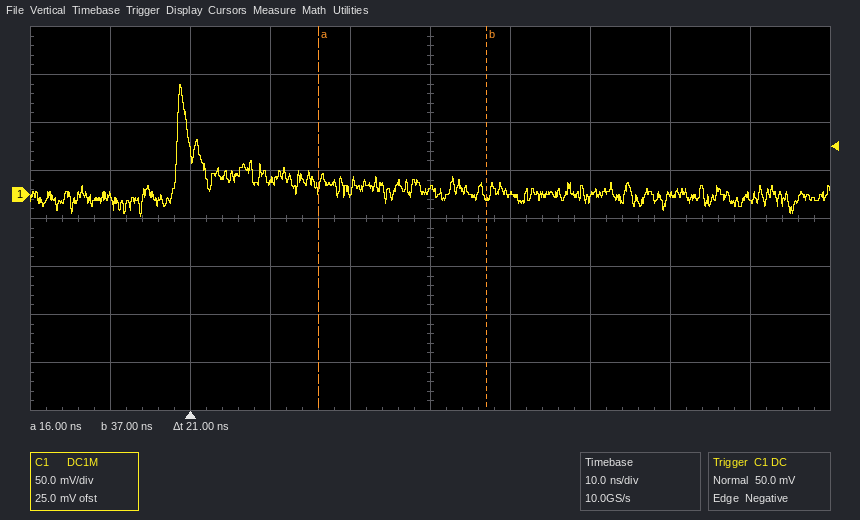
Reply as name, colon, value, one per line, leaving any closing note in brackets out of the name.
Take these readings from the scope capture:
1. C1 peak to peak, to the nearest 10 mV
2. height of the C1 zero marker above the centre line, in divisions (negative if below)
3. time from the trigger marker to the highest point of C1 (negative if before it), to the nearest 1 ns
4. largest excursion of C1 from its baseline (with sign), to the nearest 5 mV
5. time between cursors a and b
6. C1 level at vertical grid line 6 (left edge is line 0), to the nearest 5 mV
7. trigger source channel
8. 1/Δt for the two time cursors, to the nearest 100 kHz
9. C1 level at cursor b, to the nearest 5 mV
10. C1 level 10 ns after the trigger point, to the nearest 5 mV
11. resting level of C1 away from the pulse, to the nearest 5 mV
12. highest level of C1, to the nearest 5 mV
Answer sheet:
C1 peak to peak, to the nearest 10 mV: 140 mV
height of the C1 zero marker above the centre line, in divisions: +0.5 div
time from the trigger marker to the highest point of C1 (negative if before it), to the nearest 1 ns: -1 ns
largest excursion of C1 from its baseline (with sign), to the nearest 5 mV: +115 mV
time between cursors a and b: 21 ns
C1 level at vertical grid line 6 (left edge is line 0), to the nearest 5 mV: 0 mV
trigger source channel: C1
1/Δt for the two time cursors, to the nearest 100 kHz: 47.6 MHz
C1 level at cursor b, to the nearest 5 mV: -5 mV
C1 level 10 ns after the trigger point, to the nearest 5 mV: 15 mV
resting level of C1 away from the pulse, to the nearest 5 mV: 0 mV
highest level of C1, to the nearest 5 mV: 115 mV
